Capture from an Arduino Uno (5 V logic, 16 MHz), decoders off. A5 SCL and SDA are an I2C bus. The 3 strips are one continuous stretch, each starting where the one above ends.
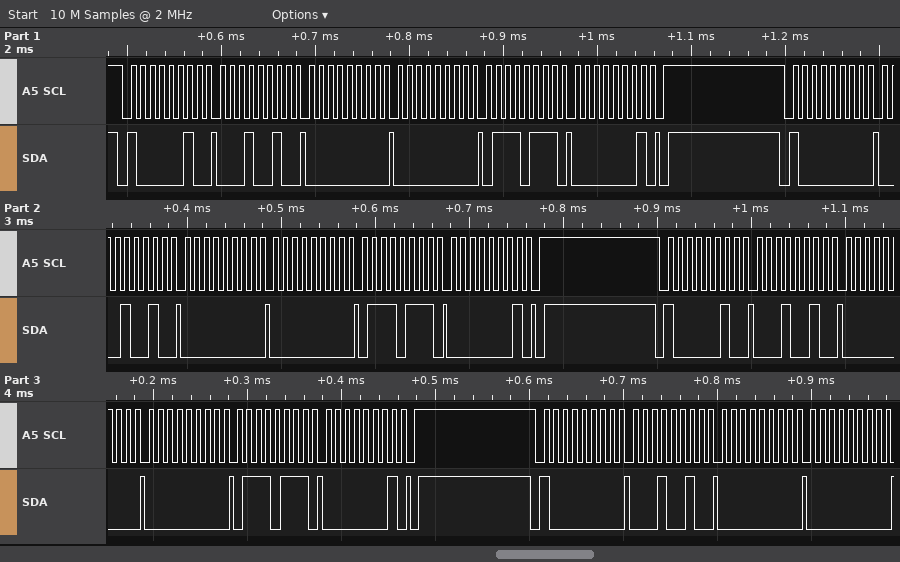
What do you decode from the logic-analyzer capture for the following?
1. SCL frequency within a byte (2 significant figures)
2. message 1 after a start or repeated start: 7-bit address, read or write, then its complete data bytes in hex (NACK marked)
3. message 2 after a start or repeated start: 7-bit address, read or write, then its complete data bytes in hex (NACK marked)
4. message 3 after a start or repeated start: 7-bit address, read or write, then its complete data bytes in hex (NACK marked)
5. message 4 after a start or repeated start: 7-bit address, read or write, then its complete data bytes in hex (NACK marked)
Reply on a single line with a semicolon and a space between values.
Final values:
100 kHz; 0x41 write: 12 00 00 77 01; 0x40 write: 12 00 00 77 01; 0x41 write: 12 00 00 77 01; 0x40 write: 12 00 00
